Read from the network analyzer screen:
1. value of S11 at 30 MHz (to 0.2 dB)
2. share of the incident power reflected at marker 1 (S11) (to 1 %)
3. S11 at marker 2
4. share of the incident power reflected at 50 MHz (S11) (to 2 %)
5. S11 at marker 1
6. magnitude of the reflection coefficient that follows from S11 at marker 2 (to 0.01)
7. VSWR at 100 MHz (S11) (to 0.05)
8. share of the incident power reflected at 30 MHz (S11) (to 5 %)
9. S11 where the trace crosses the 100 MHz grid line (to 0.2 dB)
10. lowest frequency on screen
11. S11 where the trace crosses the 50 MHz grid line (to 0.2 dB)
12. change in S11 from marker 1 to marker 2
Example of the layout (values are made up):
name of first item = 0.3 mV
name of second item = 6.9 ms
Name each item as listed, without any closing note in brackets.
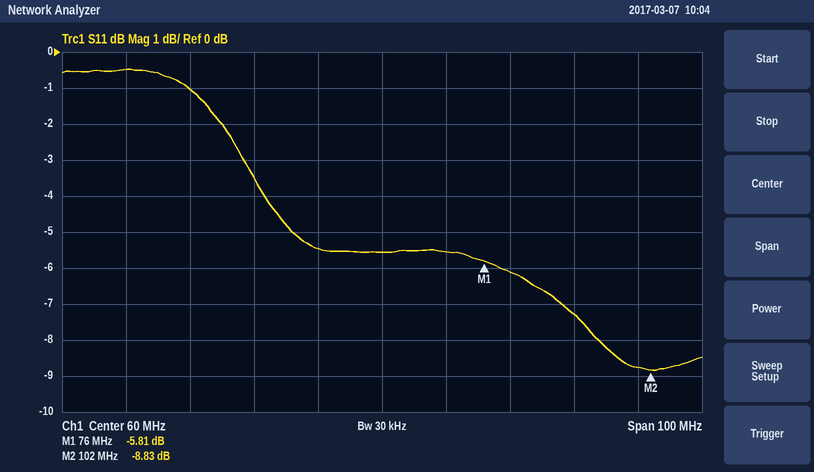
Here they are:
value of S11 at 30 MHz = -1.0 dB
share of the incident power reflected at marker 1 (S11) = 26 %
S11 at marker 2 = -8.83 dB
share of the incident power reflected at 50 MHz (S11) = 28 %
S11 at marker 1 = -5.81 dB
magnitude of the reflection coefficient that follows from S11 at marker 2 = 0.36
VSWR at 100 MHz (S11) = 2.15
share of the incident power reflected at 30 MHz (S11) = 80 %
S11 where the trace crosses the 100 MHz grid line = -8.8 dB
lowest frequency on screen = 10 MHz
S11 where the trace crosses the 50 MHz grid line = -5.4 dB
change in S11 from marker 1 to marker 2 = -3.02 dB
